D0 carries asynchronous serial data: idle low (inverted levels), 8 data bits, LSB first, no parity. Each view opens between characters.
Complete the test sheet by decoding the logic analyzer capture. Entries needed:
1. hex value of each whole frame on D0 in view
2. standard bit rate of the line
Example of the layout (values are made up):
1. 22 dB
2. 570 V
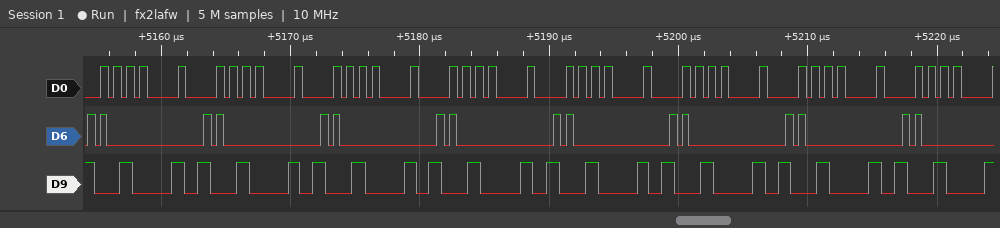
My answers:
1. D5, 5F, 7D, D5, 5F, 7D, D5, 5F, 7D, D5, 5F
2. 2000000 baud
